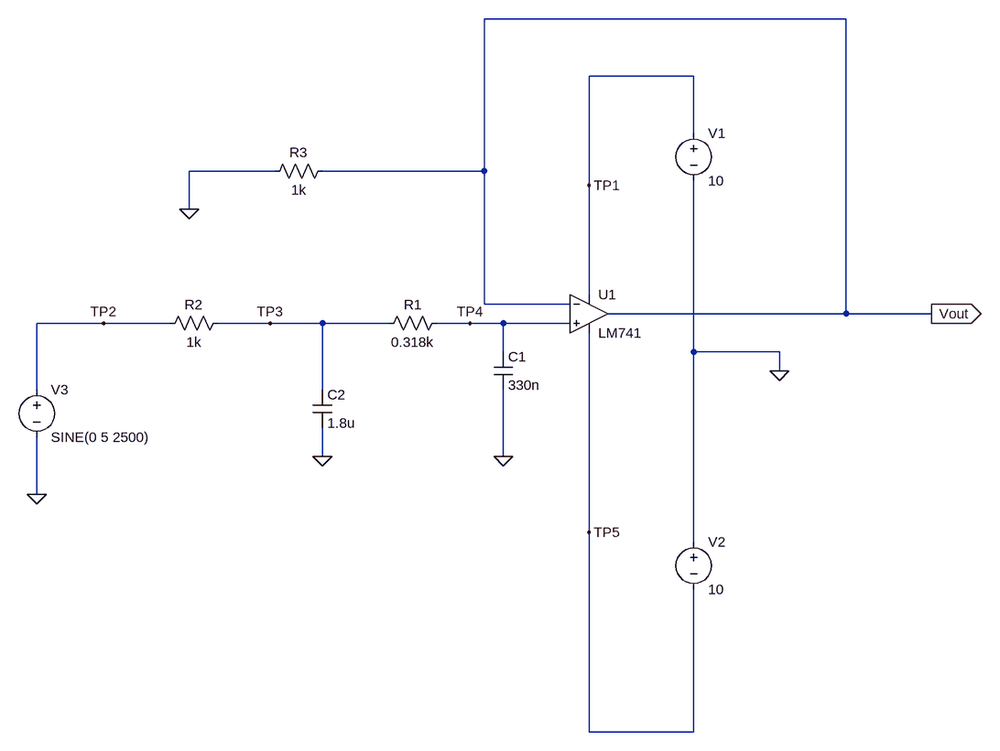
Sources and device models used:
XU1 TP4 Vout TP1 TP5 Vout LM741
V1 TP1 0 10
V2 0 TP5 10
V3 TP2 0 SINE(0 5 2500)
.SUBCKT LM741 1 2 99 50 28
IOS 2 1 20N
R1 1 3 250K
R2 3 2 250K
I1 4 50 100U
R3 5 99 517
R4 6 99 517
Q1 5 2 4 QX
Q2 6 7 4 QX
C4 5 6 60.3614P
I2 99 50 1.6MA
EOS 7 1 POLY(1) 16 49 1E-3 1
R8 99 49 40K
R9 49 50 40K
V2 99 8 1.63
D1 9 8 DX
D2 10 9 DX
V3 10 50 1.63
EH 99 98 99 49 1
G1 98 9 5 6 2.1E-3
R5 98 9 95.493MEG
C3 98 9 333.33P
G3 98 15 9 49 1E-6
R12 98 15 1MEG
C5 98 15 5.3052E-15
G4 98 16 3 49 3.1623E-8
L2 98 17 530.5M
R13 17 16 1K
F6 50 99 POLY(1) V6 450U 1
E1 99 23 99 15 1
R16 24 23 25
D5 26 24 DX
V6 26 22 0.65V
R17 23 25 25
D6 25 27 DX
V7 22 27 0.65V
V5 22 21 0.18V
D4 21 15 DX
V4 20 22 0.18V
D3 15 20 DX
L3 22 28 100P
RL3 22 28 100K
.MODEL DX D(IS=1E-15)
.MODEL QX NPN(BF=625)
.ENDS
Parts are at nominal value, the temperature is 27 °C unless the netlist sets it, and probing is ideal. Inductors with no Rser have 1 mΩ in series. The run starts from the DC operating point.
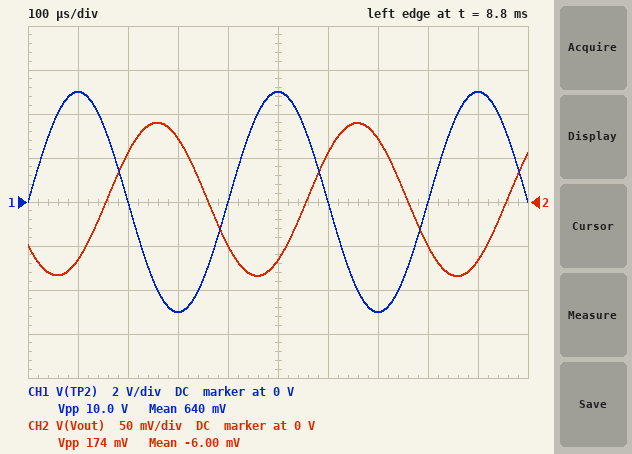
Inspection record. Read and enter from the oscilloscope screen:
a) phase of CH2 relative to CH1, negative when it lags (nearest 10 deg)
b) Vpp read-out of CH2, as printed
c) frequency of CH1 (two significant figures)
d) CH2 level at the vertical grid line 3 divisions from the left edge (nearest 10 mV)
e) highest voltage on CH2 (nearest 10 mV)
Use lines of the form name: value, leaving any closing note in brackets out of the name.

phase of CH2 relative to CH1, negative when it lags: -140 deg
Vpp read-out of CH2, as printed: 174 mV
frequency of CH1: 2.5 kHz
CH2 level at the vertical grid line 3 divisions from the left edge: 70 mV
highest voltage on CH2: 90 mV
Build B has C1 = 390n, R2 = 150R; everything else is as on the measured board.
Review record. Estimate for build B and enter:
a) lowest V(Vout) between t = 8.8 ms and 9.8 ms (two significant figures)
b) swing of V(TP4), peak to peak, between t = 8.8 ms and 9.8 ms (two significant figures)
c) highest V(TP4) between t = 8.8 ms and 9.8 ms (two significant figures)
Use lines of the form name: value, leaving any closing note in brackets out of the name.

lowest V(Vout) between t = 8.8 ms and 9.8 ms: -490 mV
swing of V(TP4), peak to peak, between t = 8.8 ms and 9.8 ms: 980 mV
highest V(TP4) between t = 8.8 ms and 9.8 ms: 490 mV
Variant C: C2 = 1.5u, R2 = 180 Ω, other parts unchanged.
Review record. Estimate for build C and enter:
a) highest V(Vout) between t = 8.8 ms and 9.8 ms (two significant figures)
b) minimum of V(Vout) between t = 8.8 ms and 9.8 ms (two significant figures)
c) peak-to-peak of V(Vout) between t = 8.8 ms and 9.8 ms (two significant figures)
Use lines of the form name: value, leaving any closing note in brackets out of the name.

highest V(Vout) between t = 8.8 ms and 9.8 ms: 550 mV
minimum of V(Vout) between t = 8.8 ms and 9.8 ms: -550 mV
peak-to-peak of V(Vout) between t = 8.8 ms and 9.8 ms: 1.1 V
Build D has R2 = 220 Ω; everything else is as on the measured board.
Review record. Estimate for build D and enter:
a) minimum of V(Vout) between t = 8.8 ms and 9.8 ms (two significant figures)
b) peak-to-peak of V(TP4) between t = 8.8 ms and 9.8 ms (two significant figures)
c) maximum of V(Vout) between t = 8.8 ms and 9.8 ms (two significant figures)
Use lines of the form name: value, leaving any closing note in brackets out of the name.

minimum of V(Vout) between t = 8.8 ms and 9.8 ms: -390 mV
peak-to-peak of V(TP4) between t = 8.8 ms and 9.8 ms: 770 mV
maximum of V(Vout) between t = 8.8 ms and 9.8 ms: 390 mV
